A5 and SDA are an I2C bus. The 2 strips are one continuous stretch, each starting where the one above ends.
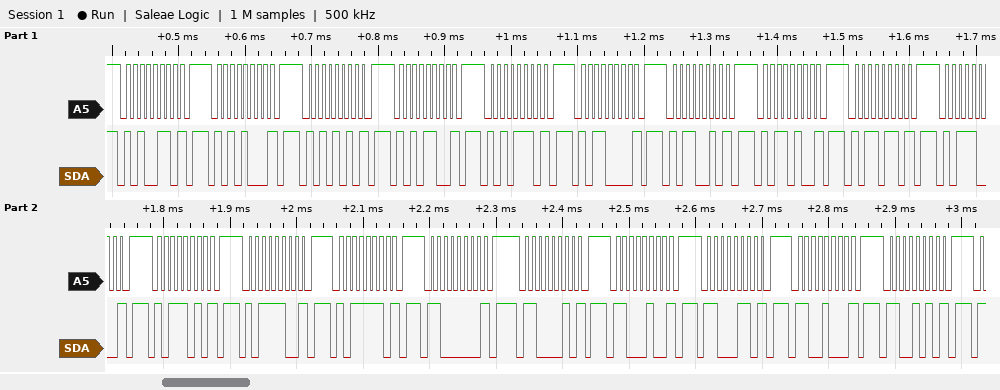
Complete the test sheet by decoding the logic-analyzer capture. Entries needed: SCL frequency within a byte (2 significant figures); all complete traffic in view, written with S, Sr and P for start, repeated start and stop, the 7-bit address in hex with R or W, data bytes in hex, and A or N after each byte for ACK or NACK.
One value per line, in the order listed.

100 kHz
S 53W N P S 54W N P S 55W N P S 56W N P S 57W N P S 58W N P S 59W N P S 5AW N P S 5BW N P S 5CW N P S 5DW N P S 5EW N P S 5FW N P S 60W N P S 61W N P S 62W N P S 63W N P S 64W N P S 65W N P
